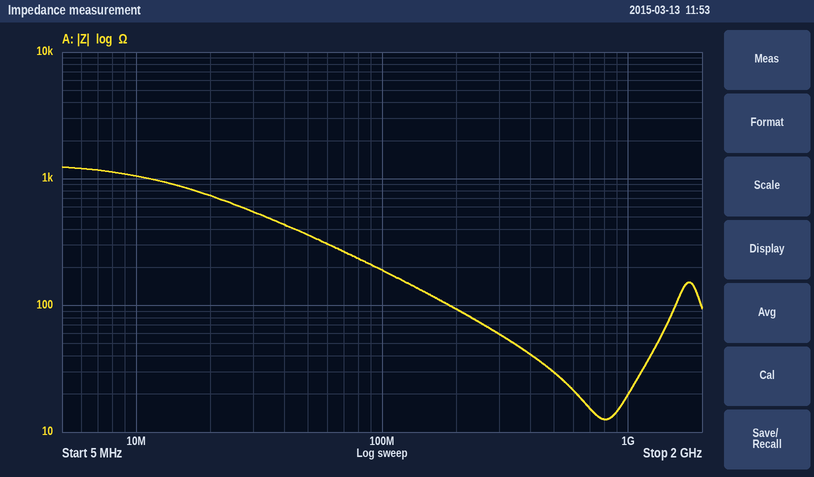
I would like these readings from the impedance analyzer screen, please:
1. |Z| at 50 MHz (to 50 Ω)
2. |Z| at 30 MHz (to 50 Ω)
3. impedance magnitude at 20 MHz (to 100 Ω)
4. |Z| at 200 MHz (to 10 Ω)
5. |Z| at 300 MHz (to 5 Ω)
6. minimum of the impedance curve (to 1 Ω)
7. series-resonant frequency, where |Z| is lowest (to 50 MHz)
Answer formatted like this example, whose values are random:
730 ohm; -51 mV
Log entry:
350 Ω; 550 Ω; 700 Ω; 90 Ω; 60 Ω; 13 Ω; 800 MHz
